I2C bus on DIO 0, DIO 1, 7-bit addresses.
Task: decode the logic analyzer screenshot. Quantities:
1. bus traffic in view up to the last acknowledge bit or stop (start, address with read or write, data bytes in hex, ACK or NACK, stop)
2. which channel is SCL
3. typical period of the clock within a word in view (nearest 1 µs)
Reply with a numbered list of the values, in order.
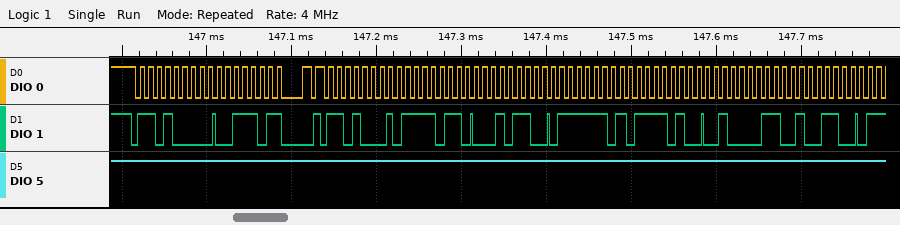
1. start, address 68 write ACK, 3B ACK, repeated start, address 68 read ACK, F6 ACK, 2C ACK, FD ACK, F4 ACK, 43 ACK, 4C ACK
2. DIO 0
3. 10 µs
